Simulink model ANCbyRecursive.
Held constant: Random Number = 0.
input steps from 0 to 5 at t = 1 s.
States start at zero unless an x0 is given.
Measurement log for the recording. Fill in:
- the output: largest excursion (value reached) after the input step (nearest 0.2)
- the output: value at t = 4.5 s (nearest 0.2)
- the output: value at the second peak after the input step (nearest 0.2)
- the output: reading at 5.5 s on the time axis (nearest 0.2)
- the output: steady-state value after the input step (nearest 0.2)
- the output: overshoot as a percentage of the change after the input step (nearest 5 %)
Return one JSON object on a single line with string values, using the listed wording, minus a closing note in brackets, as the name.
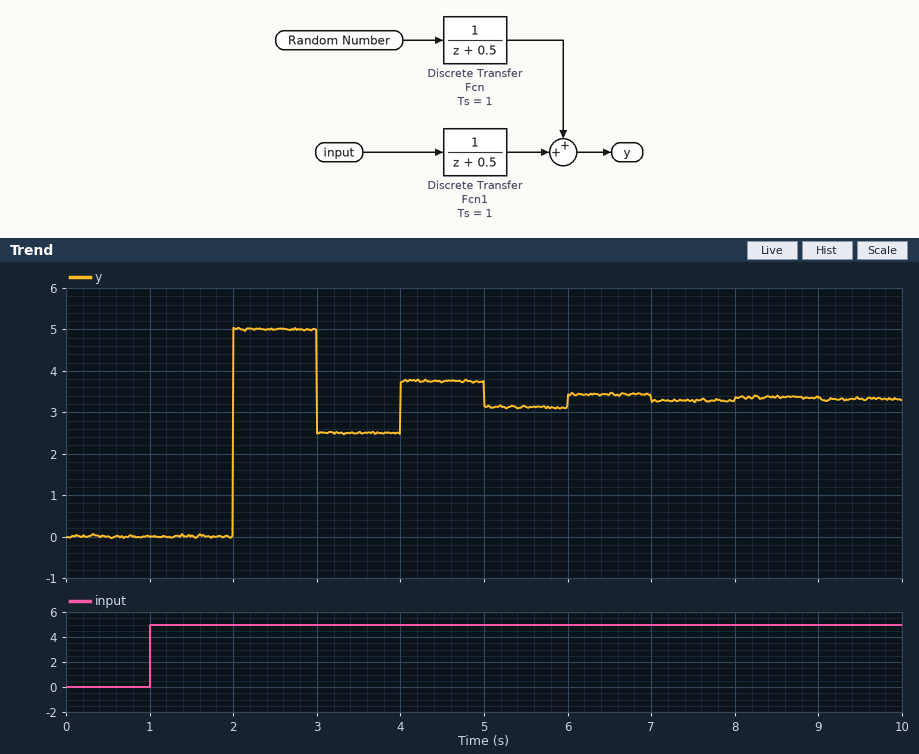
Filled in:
{"the output: largest excursion (value reached) after the input step": "5.0", "the output: value at t = 4.5 s": "3.8", "the output: value at the second peak after the input step": "3.8", "the output: reading at 5.5 s on the time axis": "3.2", "the output: steady-state value after the input step": "3.4", "the output: overshoot as a percentage of the change after the input step": "50 %"}
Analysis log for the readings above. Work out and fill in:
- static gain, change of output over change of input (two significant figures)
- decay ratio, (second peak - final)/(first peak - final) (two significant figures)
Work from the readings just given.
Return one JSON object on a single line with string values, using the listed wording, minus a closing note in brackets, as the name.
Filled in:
{"static gain, change of output over change of input": "0.68", "decay ratio, (second peak - final)/(first peak - final)": "0.25"}
